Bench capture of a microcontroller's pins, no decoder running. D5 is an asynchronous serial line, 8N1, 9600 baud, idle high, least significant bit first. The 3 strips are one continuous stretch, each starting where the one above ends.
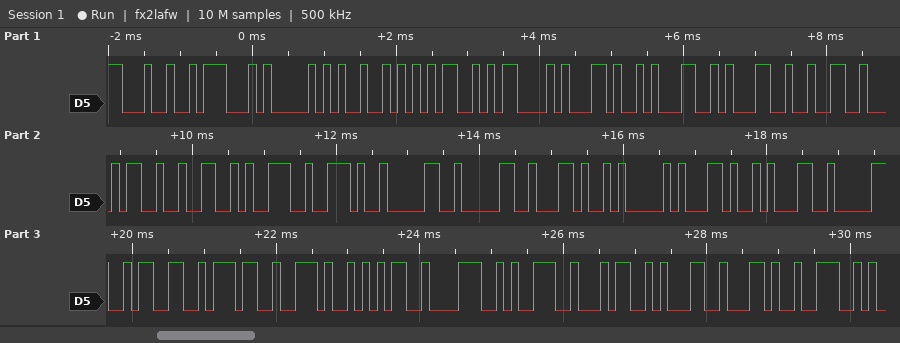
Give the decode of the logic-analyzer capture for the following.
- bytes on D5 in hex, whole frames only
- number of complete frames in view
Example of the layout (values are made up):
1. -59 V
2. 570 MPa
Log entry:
1. 24 47 50 52 4D 43 2C 31 31 32 34 32 39 2E 30 30 2C 41 2C 31 30 33 37 2E 35 38 39 34 31 2C 4E
2. 31
